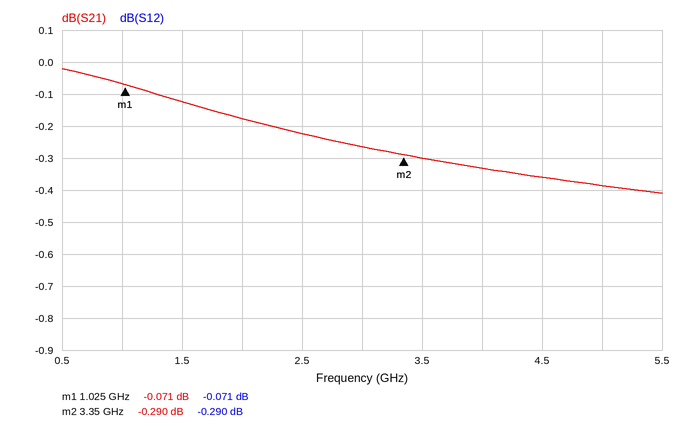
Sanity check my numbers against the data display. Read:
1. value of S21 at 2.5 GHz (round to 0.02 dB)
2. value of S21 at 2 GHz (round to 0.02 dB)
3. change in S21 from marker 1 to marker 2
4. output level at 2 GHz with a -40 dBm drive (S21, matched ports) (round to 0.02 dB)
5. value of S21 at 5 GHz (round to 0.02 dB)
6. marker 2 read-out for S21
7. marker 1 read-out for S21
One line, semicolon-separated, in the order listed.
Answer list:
-0.22 dB; -0.18 dB; -0.219 dB; -40.18 dBm; -0.38 dB; -0.290 dB; -0.071 dB
